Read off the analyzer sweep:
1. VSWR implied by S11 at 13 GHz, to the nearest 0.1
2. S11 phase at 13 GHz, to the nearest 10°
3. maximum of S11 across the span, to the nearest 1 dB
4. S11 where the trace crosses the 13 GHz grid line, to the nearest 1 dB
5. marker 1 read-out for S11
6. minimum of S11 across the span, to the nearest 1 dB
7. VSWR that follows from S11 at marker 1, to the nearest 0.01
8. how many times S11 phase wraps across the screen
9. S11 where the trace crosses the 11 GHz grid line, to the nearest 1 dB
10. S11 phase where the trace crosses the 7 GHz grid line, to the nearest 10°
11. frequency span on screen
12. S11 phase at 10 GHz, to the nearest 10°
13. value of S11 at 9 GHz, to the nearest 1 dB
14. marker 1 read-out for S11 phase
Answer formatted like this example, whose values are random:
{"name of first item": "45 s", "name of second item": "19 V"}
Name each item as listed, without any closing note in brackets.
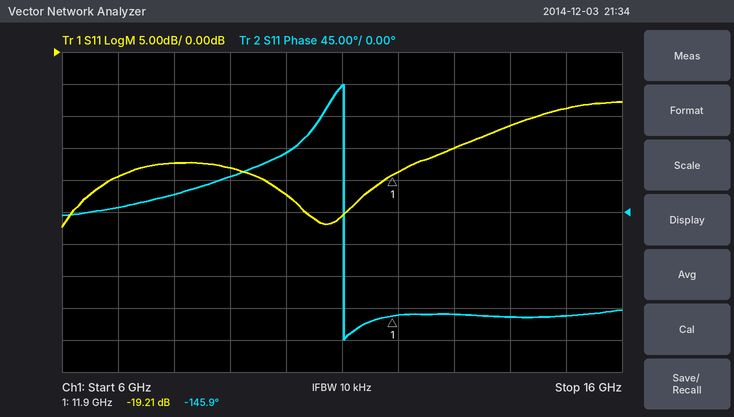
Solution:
{"VSWR implied by S11 at 13 GHz, to the nearest 0.1": "1.4", "S11 phase at 13 GHz, to the nearest 10°": "-140°", "maximum of S11 across the span, to the nearest 1 dB": "-8 dB", "S11 where the trace crosses the 13 GHz grid line, to the nearest 1 dB": "-15 dB", "marker 1 read-out for S11": "-19.21 dB", "minimum of S11 across the span, to the nearest 1 dB": "-27 dB", "VSWR that follows from S11 at marker 1, to the nearest 0.01": "1.25", "how many times S11 phase wraps across the screen": "1", "S11 where the trace crosses the 11 GHz grid line, to the nearest 1 dB": "-26 dB", "S11 phase where the trace crosses the 7 GHz grid line, to the nearest 10°": "10°", "frequency span on screen": "10 GHz", "S11 phase at 10 GHz, to the nearest 10°": "80°", "value of S11 at 9 GHz, to the nearest 1 dB": "-18 dB", "marker 1 read-out for S11 phase": "-145.9°"}
